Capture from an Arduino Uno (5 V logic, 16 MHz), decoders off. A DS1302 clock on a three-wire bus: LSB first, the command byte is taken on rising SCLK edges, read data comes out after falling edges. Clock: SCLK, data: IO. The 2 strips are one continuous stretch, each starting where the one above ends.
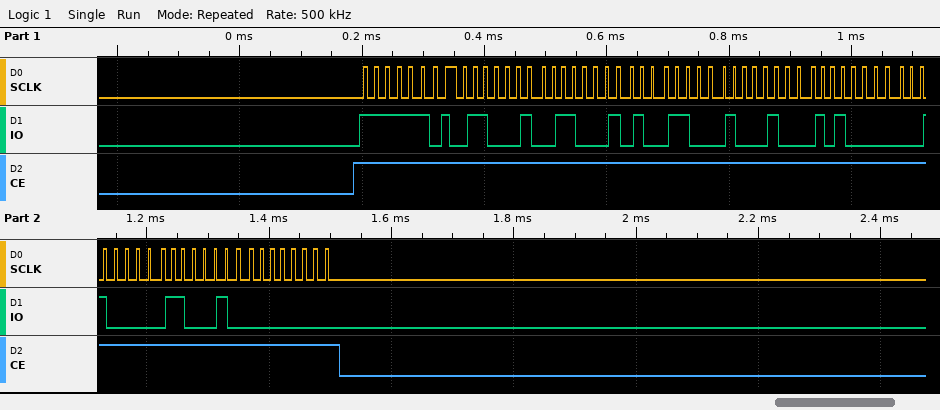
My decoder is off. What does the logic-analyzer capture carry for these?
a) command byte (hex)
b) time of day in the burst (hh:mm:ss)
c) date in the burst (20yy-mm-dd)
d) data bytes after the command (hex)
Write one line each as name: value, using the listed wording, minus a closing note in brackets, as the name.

command byte: 0xBF
time of day in the burst: 19:46:46
date in the burst: 2023-05-11
data bytes after the command: 46 46 19 11 05 04 23 00
